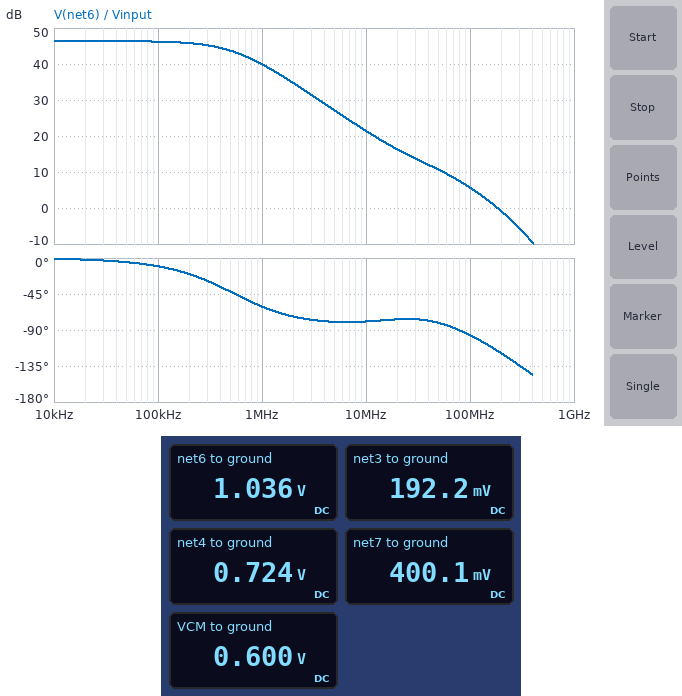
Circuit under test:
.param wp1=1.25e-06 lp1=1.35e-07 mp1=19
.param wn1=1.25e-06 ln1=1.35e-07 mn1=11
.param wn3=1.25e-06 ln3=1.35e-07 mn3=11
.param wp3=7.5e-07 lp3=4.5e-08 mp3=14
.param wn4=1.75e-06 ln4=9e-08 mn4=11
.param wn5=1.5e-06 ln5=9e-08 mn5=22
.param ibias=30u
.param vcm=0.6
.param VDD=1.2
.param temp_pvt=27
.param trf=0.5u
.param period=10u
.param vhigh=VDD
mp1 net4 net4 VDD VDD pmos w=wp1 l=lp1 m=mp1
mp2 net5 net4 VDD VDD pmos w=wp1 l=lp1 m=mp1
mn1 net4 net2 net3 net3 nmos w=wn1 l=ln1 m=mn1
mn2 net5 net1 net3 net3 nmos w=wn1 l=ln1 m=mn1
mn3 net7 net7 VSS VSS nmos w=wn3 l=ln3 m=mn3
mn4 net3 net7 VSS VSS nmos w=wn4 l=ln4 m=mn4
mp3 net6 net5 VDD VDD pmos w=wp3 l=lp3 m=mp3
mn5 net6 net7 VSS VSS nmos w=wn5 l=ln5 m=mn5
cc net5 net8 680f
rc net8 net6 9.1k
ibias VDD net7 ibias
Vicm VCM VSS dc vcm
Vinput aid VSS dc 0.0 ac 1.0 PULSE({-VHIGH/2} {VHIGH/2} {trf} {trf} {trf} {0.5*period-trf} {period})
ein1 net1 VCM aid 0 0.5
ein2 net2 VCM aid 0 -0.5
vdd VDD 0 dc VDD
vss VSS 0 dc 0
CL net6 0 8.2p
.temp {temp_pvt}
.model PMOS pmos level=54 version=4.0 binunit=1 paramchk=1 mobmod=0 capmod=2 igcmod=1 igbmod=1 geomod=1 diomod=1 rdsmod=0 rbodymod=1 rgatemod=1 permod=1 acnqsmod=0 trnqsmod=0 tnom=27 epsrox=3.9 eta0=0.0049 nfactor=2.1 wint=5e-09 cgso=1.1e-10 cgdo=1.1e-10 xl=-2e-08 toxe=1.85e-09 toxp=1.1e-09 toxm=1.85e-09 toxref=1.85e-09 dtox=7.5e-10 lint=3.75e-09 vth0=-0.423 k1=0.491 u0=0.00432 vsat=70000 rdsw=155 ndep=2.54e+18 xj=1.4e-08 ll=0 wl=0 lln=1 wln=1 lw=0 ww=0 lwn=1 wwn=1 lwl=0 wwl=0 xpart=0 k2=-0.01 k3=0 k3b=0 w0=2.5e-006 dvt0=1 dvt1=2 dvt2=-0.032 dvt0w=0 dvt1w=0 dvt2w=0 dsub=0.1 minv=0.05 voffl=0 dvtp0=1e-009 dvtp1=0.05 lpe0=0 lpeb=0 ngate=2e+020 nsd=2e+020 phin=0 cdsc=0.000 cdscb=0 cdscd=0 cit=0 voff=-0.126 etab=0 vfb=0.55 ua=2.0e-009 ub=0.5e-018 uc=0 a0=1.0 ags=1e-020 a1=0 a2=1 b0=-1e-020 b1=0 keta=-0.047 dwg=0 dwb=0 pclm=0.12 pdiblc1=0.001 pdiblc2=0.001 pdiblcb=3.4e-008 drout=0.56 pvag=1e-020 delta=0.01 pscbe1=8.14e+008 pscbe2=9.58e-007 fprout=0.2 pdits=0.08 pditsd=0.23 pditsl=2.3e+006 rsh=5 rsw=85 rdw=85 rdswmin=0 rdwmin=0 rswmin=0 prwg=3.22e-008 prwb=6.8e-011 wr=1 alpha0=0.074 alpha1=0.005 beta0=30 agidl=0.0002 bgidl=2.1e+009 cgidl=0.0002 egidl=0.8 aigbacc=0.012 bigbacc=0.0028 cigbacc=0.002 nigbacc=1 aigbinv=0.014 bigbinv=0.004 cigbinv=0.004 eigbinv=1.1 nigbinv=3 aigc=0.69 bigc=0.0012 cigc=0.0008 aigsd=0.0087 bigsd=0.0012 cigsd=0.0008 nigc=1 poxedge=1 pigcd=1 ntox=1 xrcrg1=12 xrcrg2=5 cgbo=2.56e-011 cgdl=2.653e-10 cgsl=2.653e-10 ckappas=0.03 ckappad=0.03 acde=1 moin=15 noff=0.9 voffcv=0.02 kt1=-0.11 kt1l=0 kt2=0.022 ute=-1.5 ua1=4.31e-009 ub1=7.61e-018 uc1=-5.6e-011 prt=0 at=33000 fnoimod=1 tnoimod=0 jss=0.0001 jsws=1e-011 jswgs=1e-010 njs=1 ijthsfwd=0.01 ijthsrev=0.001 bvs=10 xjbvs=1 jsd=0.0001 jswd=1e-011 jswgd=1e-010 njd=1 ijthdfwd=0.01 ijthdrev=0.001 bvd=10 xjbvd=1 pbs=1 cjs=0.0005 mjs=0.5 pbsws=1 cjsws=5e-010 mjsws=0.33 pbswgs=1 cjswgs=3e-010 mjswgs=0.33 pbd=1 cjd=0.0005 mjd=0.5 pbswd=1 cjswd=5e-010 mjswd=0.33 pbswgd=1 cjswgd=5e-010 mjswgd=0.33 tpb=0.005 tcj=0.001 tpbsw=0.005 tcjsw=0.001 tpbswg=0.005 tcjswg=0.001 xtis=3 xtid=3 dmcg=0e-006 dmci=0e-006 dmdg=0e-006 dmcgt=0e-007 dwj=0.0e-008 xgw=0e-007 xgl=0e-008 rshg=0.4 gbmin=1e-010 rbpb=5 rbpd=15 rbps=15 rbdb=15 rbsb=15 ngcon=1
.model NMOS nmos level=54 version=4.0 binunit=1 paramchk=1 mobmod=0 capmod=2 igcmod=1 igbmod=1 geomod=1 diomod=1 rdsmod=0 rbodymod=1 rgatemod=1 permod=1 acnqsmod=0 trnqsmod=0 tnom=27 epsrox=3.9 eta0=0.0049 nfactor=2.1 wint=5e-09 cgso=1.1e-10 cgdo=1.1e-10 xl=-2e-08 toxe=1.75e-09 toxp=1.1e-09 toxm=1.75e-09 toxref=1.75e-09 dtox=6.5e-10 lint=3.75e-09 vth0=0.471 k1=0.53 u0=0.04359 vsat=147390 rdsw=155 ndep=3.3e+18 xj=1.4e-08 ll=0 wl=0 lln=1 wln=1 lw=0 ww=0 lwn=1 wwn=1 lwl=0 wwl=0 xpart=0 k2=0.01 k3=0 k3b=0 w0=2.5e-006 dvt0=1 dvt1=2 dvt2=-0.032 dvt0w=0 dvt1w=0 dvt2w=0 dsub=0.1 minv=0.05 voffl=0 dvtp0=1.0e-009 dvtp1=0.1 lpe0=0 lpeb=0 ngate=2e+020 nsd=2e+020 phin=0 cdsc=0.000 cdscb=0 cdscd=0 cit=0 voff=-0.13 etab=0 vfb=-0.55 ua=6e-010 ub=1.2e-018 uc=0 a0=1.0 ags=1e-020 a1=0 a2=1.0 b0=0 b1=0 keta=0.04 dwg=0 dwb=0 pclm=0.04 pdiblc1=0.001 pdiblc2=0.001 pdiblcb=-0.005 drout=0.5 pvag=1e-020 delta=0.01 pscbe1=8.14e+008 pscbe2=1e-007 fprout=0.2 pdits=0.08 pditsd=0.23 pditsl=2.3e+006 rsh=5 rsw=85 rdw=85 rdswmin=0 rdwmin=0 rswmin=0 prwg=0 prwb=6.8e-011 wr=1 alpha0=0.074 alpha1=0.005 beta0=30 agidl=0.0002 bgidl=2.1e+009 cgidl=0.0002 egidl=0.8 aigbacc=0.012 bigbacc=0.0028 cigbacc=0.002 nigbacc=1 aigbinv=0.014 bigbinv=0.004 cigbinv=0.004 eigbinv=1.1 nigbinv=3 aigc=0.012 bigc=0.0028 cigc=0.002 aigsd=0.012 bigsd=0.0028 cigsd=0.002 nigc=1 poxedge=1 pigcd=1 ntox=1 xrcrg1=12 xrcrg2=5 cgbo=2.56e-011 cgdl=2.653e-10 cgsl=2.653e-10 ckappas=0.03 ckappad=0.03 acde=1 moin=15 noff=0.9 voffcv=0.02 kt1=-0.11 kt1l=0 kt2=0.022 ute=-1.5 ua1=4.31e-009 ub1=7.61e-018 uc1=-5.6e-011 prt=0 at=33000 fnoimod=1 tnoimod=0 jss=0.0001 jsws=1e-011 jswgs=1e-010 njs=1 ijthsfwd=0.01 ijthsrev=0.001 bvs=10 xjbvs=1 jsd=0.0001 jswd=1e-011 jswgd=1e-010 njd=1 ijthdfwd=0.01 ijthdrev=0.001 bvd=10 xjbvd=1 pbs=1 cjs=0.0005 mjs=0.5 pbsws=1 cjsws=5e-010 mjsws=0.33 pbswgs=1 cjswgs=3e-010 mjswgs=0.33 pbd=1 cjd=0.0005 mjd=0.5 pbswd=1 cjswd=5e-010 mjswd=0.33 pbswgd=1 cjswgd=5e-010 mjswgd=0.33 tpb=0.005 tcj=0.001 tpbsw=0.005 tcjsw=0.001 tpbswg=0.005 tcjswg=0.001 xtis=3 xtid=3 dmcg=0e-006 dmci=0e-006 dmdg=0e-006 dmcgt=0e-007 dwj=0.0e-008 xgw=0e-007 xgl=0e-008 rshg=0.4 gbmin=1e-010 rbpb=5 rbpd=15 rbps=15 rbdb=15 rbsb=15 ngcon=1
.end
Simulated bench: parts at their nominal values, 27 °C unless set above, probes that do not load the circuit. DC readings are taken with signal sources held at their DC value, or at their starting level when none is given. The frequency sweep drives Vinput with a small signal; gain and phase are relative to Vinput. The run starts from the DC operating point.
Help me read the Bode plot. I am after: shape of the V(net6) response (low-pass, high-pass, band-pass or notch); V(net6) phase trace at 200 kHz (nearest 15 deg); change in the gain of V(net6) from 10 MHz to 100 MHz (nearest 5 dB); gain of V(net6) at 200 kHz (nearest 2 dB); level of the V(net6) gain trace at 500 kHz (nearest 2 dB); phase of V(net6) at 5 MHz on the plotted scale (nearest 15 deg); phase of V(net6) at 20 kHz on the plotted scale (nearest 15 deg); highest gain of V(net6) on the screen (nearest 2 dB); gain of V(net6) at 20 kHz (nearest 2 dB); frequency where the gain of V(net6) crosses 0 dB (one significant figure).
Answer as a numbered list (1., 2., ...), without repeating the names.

1. low-pass
2. -15 deg
3. -15 dB
4. 46 dB
5. 44 dB
6. -75 deg
7. 0 deg
8. 46 dB
9. 46 dB
10. 200 MHz
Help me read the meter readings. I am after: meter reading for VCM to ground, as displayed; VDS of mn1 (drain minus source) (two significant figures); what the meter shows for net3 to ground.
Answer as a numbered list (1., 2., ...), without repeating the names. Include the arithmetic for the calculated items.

1. 0.600 V
2. 724 mV - 192.2 mV = 530 mV
3. 192.2 mV
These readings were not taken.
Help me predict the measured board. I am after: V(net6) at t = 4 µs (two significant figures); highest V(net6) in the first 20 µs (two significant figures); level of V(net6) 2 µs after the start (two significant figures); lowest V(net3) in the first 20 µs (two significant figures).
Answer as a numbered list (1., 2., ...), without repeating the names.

1. 1.2 V
2. 1.2 V
3. 1.2 V
4. 4.1 mV
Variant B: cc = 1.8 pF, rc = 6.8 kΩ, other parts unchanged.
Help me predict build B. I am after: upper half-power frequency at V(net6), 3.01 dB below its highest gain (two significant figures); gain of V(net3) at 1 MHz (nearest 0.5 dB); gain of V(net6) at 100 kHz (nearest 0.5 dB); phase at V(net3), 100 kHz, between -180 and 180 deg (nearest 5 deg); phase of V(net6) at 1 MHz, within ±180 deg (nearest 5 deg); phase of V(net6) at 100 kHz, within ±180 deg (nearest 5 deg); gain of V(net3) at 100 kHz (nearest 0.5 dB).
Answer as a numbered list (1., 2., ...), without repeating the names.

1. 210 kHz
2. -25.0 dB
3. 45.5 dB
4. 155 deg
5. -75 deg
6. -25 deg
7. -12.5 dB
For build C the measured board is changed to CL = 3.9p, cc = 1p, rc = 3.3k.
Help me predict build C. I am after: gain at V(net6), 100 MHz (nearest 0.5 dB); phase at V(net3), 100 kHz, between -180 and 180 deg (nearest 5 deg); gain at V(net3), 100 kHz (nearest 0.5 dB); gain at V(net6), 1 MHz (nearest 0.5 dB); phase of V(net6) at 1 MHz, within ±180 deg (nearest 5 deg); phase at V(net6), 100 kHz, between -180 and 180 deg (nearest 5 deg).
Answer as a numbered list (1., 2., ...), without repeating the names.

1. 1.5 dB
2. 165 deg
3. -12.0 dB
4. 37.5 dB
5. -70 deg
6. -15 deg
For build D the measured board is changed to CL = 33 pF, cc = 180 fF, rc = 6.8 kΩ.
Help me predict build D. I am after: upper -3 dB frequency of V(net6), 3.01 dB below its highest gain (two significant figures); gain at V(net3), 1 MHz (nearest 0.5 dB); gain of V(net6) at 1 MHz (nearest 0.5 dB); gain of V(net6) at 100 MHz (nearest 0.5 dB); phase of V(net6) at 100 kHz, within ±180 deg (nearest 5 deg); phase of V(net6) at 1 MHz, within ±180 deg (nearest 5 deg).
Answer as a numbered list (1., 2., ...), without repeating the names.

1. 1.3 MHz
2. -13.0 dB
3. 44.5 dB
4. -5.5 dB
5. -5 deg
6. -40 deg
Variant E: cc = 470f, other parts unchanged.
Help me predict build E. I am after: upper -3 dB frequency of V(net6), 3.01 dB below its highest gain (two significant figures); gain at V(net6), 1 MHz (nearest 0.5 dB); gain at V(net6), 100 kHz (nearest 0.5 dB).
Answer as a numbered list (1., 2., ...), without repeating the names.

1. 770 kHz
2. 42.0 dB
3. 46.5 dB
